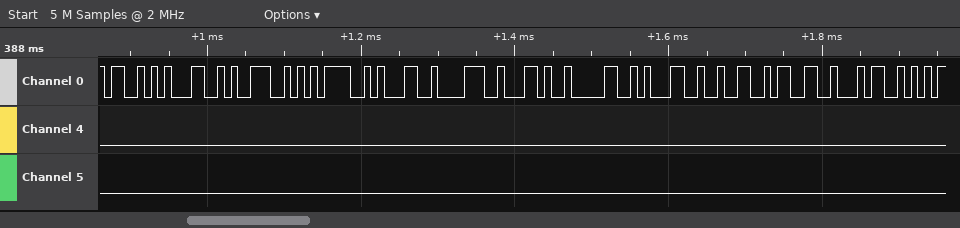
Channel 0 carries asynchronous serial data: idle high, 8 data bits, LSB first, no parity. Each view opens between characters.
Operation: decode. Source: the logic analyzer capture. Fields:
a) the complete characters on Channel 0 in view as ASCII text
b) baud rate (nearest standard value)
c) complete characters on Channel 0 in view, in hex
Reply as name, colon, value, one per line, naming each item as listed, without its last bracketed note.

the complete characters on Channel 0 in view as ASCII text: "SLN=18,01234"
baud rate: 115200 baud
complete characters on Channel 0 in view, in hex: 53, 4C, 4E, 3D, 31, 38, 2C, 30, 31, 32, 33, 34
